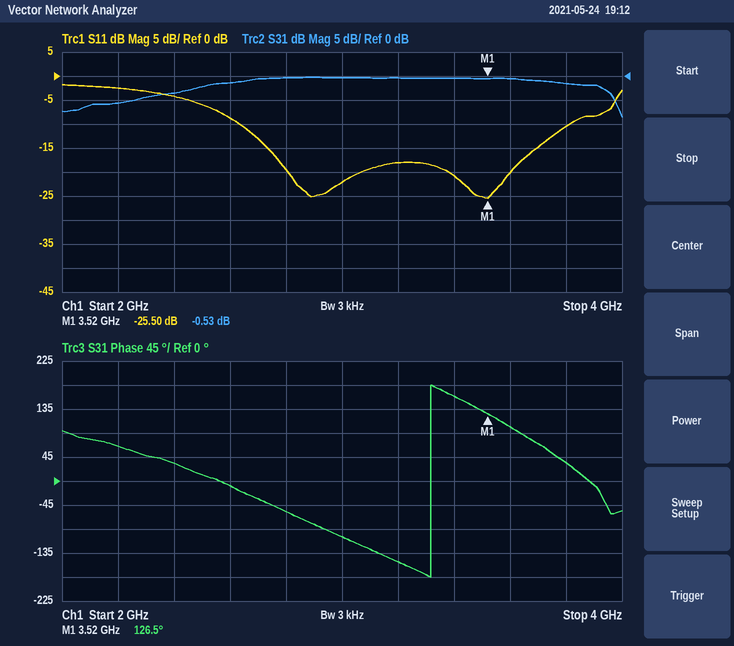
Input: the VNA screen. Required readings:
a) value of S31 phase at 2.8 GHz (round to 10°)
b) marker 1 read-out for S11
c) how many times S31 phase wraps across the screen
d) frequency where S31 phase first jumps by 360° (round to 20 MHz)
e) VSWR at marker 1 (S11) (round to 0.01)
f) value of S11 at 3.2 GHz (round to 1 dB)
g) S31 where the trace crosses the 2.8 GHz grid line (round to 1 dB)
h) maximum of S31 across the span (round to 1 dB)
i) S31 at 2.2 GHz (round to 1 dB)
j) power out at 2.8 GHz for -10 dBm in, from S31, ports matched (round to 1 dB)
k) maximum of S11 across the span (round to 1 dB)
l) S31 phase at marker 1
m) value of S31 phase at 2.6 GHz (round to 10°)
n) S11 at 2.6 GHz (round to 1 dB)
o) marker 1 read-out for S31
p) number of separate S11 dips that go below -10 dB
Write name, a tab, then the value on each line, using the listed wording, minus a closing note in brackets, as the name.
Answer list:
value of S31 phase at 2.8 GHz	-60°
marker 1 read-out for S11	-25.50 dB
how many times S31 phase wraps across the screen	1
frequency where S31 phase first jumps by 360°	3.32 GHz
VSWR at marker 1 (S11)	1.11
value of S11 at 3.2 GHz	-18 dB
S31 where the trace crosses the 2.8 GHz grid line	0 dB
maximum of S31 across the span	0 dB
S31 at 2.2 GHz	-6 dB
power out at 2.8 GHz for -10 dBm in, from S31, ports matched	-10 dBm
maximum of S11 across the span	-2 dB
S31 phase at marker 1	126.5°
value of S31 phase at 2.6 GHz	-10°
S11 at 2.6 GHz	-9 dB
marker 1 read-out for S31	-0.53 dB
number of separate S11 dips that go below -10 dB	2
